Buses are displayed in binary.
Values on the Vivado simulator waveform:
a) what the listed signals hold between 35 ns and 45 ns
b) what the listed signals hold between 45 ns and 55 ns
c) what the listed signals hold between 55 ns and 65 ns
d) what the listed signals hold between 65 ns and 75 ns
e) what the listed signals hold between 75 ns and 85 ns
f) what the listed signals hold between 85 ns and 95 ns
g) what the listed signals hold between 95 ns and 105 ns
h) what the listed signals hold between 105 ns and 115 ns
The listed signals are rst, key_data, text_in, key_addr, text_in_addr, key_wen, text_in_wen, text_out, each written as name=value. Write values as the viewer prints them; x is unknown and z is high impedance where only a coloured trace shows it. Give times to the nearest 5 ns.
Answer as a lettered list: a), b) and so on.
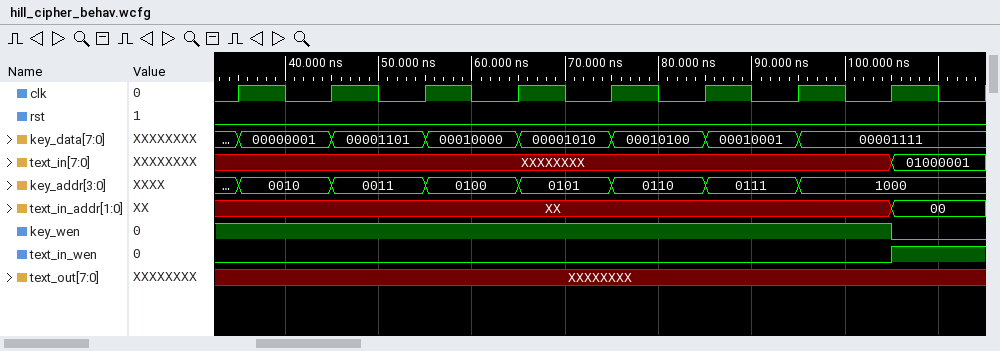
a) rst=0, key_data=00000001, text_in=XXXXXXXX, key_addr=0010, text_in_addr=XX, key_wen=1, text_in_wen=0, text_out=XXXXXXXX
b) rst=0, key_data=00001101, text_in=XXXXXXXX, key_addr=0011, text_in_addr=XX, key_wen=1, text_in_wen=0, text_out=XXXXXXXX
c) rst=0, key_data=00010000, text_in=XXXXXXXX, key_addr=0100, text_in_addr=XX, key_wen=1, text_in_wen=0, text_out=XXXXXXXX
d) rst=0, key_data=00001010, text_in=XXXXXXXX, key_addr=0101, text_in_addr=XX, key_wen=1, text_in_wen=0, text_out=XXXXXXXX
e) rst=0, key_data=00010100, text_in=XXXXXXXX, key_addr=0110, text_in_addr=XX, key_wen=1, text_in_wen=0, text_out=XXXXXXXX
f) rst=0, key_data=00010001, text_in=XXXXXXXX, key_addr=0111, text_in_addr=XX, key_wen=1, text_in_wen=0, text_out=XXXXXXXX
g) rst=0, key_data=00001111, text_in=XXXXXXXX, key_addr=1000, text_in_addr=XX, key_wen=1, text_in_wen=0, text_out=XXXXXXXX
h) rst=0, key_data=00001111, text_in=01000001, key_addr=1000, text_in_addr=00, key_wen=0, text_in_wen=1, text_out=XXXXXXXX
